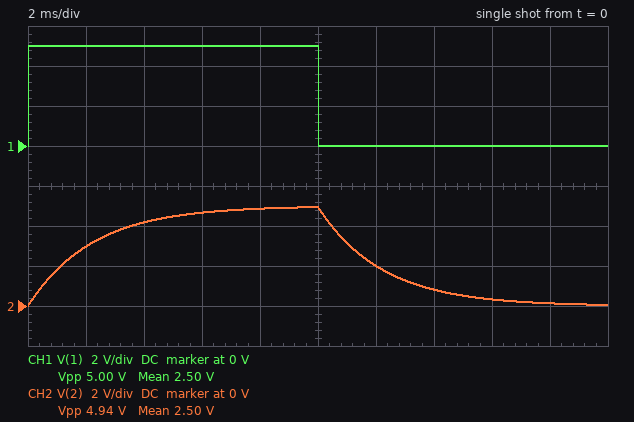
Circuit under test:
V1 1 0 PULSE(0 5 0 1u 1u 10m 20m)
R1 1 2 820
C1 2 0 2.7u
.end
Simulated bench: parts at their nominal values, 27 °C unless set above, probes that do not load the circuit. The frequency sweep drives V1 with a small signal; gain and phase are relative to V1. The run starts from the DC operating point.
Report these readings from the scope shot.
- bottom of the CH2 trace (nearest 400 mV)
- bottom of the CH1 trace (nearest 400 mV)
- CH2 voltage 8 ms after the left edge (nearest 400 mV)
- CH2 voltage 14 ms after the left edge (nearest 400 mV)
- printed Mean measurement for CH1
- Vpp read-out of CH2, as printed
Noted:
0 V
0 V
4.8 V
800 mV
2.50 V
4.94 V
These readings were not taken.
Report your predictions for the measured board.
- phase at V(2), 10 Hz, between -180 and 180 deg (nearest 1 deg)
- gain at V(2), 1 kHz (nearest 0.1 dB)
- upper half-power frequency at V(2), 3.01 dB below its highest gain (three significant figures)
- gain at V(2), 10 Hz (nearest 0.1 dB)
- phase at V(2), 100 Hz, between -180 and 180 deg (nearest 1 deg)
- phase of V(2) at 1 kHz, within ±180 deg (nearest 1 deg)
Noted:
-8 deg
-22.9 dB
71.9 Hz
-0.1 dB
-54 deg
-86 deg
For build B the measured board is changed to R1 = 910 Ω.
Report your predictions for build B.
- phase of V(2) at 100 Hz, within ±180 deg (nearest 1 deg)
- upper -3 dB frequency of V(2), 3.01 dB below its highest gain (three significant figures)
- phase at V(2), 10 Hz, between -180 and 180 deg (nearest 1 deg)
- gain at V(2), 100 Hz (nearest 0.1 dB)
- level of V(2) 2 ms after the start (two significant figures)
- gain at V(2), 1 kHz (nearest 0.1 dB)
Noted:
-57 deg
64.8 Hz
-9 deg
-5.3 dB
2.8 V
-23.8 dB
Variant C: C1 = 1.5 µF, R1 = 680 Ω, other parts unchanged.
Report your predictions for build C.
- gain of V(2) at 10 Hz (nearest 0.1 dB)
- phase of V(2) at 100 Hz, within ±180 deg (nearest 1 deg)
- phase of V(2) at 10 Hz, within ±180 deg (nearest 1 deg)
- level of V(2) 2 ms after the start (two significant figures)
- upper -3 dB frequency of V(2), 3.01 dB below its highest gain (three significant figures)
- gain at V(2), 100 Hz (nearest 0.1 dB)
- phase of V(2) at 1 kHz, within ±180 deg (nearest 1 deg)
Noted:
0 dB
-33 deg
-4 deg
4.3 V
156 Hz
-1.5 dB
-81 deg
